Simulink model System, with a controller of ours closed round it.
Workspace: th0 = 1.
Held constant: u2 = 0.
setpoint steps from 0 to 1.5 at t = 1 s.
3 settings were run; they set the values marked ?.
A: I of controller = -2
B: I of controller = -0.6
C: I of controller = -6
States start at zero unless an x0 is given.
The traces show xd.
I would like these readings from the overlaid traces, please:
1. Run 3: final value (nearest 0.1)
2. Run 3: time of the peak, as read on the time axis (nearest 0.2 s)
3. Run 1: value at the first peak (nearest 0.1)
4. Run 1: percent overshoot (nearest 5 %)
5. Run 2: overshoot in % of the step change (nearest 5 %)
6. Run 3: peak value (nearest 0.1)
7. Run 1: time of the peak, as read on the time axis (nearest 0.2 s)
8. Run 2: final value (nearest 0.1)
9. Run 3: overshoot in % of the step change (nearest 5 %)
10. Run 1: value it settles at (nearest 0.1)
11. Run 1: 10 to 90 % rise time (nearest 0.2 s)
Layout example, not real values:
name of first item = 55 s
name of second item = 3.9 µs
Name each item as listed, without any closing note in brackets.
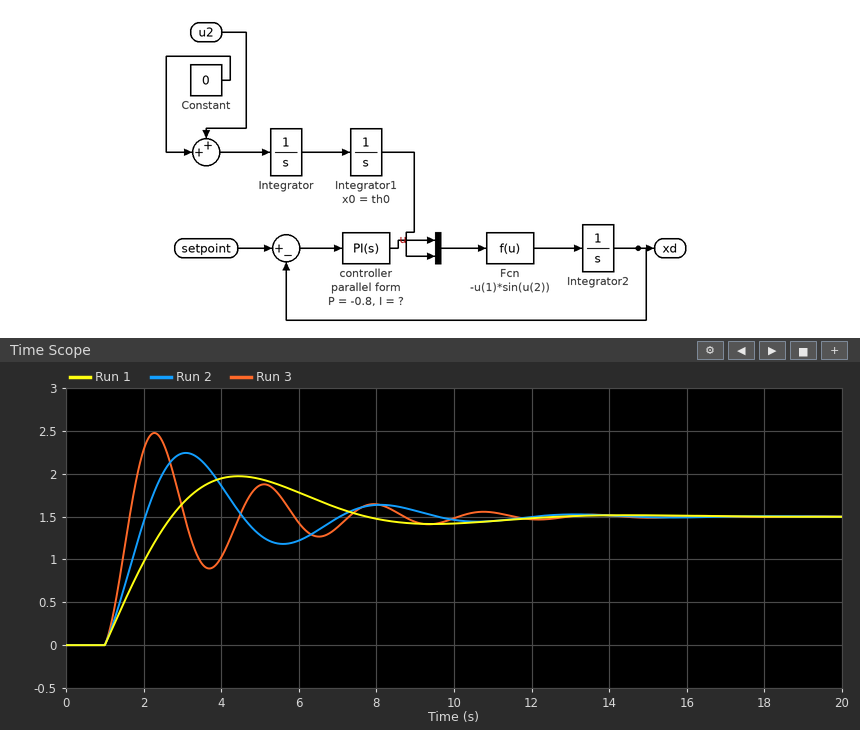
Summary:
Run 3: final value = 1.5
Run 3: time of the peak, as read on the time axis = 2.2 s
Run 1: value at the first peak = 2.0
Run 1: percent overshoot = 30 %
Run 2: overshoot in % of the step change = 50 %
Run 3: peak value = 2.5
Run 1: time of the peak, as read on the time axis = 4.4 s
Run 2: final value = 1.5
Run 3: overshoot in % of the step change = 65 %
Run 1: value it settles at = 1.5
Run 1: 10 to 90 % rise time = 1.4 s
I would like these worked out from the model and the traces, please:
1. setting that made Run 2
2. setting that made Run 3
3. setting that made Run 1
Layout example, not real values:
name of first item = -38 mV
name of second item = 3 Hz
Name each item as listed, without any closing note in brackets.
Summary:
setting that made Run 2 = A
setting that made Run 3 = C
setting that made Run 1 = B
